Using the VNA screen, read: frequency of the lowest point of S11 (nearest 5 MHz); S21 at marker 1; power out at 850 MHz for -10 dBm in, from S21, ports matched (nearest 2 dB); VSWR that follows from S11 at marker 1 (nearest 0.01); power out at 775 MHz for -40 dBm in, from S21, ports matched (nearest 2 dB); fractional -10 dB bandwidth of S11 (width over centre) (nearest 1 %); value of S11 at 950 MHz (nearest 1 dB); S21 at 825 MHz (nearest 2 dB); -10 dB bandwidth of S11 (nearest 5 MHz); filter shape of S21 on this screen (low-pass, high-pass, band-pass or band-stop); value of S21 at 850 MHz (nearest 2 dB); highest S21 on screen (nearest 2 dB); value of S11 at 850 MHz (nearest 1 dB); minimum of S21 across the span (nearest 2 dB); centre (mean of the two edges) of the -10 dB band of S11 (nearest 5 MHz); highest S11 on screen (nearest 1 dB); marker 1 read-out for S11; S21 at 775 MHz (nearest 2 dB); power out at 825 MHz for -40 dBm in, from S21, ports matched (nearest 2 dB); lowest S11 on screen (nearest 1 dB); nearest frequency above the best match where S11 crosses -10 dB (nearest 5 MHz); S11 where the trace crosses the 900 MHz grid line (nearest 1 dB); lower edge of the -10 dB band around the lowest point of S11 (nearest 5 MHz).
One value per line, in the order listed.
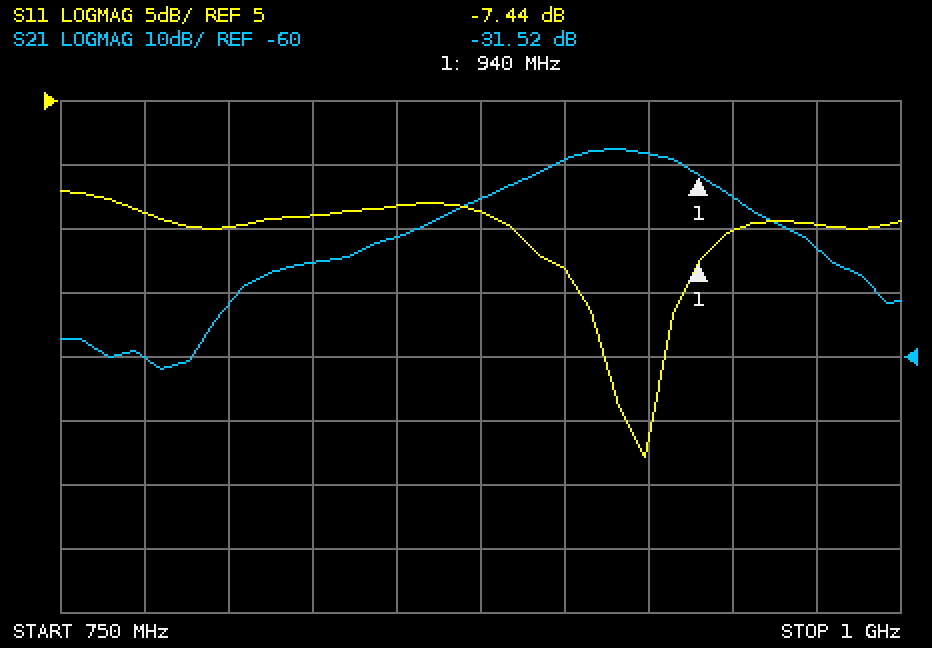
925 MHz
-31.52 dB
-52 dBm
2.48
-100 dBm
3 %
-5 dB
-46 dB
30 MHz
band-pass
-42 dB
-28 dB
-3 dB
-62 dB
920 MHz
-2 dB
-7.44 dB
-60 dB
-86 dBm
-23 dB
935 MHz
-8 dB
905 MHz
